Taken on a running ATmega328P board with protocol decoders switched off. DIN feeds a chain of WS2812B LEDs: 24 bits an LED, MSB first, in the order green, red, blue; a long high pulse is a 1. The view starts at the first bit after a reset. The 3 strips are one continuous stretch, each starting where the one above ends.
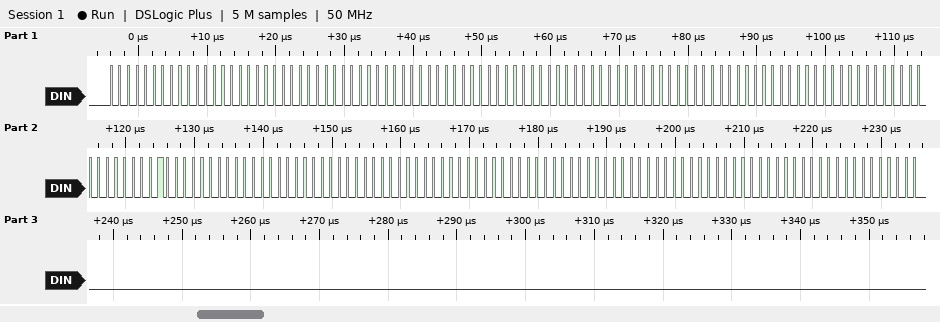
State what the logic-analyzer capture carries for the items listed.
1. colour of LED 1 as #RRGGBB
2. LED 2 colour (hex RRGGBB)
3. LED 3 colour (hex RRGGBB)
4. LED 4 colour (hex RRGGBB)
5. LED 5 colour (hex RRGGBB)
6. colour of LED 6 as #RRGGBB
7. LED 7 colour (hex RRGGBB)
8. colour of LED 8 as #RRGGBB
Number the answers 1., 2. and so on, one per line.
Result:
1. #000000
2. #000000
3. #000000
4. #000000
5. #000100
6. #000000
7. #000000
8. #000000
